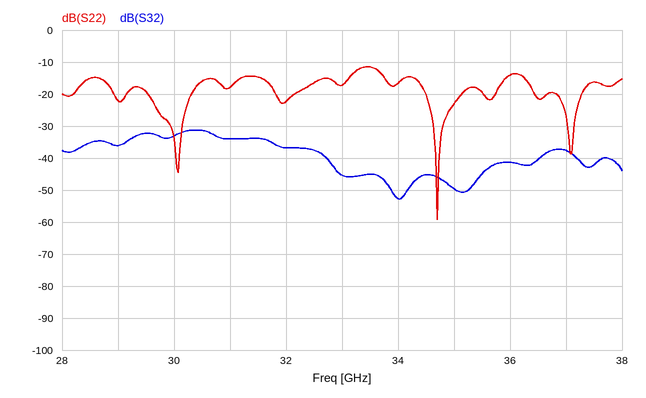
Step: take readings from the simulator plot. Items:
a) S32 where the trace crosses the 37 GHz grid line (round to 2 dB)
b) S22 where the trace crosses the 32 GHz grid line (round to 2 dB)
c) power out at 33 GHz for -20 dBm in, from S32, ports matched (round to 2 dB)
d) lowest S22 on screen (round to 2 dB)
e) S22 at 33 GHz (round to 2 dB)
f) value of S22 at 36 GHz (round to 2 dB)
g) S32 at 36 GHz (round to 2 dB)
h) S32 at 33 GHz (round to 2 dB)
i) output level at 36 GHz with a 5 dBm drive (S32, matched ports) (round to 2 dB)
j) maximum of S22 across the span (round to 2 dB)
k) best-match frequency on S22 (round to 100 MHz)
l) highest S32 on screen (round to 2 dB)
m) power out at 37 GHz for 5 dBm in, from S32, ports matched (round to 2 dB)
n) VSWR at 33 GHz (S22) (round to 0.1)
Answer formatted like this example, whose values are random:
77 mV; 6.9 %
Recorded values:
-38 dB; -22 dB; -66 dBm; -60 dB; -18 dB; -14 dB; -42 dB; -46 dB; -36 dBm; -12 dB; 34.7 GHz; -32 dB; -32 dBm; 1.3
